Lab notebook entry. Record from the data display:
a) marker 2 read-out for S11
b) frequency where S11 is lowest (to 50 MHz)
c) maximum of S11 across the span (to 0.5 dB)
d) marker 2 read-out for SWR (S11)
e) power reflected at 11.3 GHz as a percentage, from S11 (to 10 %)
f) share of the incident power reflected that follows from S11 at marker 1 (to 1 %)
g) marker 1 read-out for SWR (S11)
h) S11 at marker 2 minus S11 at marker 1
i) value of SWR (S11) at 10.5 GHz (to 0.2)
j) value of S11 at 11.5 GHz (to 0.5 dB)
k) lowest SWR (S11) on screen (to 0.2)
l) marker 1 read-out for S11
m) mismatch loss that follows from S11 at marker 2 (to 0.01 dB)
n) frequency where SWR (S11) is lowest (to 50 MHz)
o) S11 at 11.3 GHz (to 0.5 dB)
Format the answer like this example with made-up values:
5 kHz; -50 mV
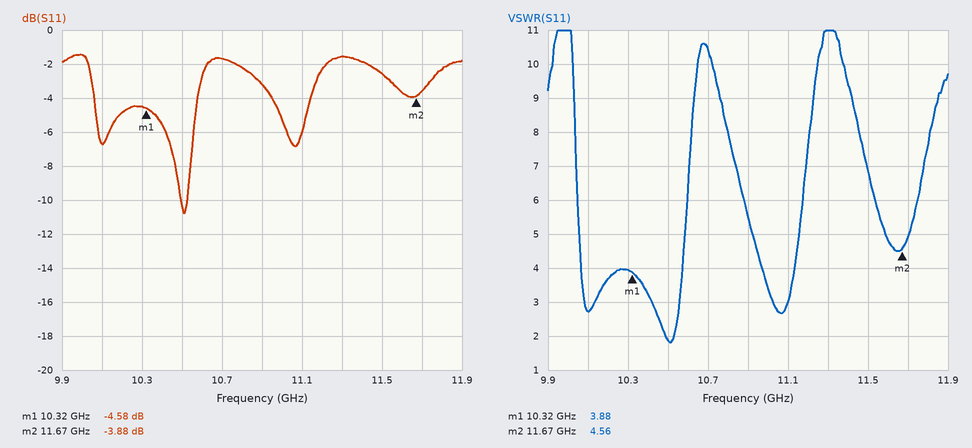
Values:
-3.88 dB; 10.50 GHz; -1.5 dB; 4.56; 70 %; 35 %; 3.88; 0.70 dB; 1.8; -2.5 dB; 1.8; -4.58 dB; 2.29 dB; 10.50 GHz; -1.5 dB
